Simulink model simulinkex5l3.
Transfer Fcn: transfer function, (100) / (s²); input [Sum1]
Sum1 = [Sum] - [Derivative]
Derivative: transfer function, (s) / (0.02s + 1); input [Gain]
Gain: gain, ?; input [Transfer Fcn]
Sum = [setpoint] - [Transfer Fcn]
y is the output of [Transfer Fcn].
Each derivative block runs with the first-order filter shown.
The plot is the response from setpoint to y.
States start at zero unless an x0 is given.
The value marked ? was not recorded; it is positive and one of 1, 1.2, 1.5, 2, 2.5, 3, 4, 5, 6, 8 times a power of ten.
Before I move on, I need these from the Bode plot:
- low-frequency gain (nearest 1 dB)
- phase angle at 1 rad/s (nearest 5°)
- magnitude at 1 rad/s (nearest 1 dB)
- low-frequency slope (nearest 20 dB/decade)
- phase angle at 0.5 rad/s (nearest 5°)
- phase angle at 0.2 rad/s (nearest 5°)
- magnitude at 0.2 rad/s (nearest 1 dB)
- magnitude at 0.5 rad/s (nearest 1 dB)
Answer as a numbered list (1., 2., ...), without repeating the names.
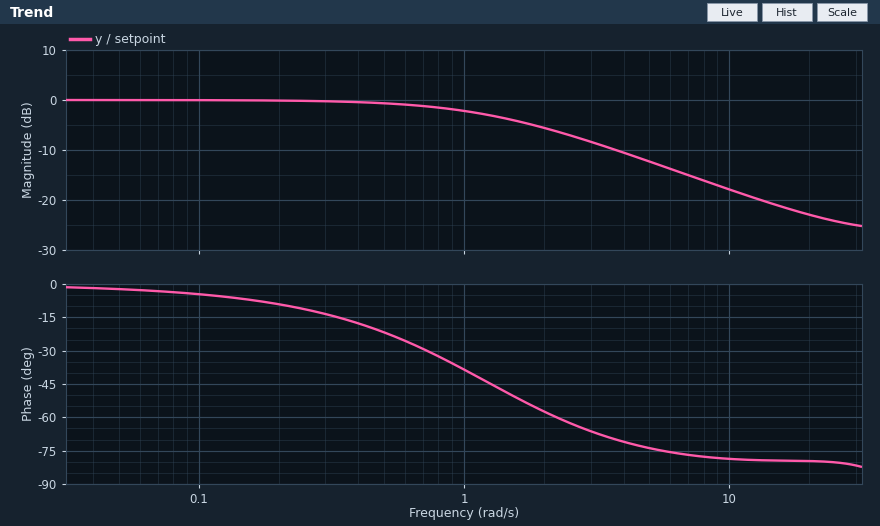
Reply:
1. 0 dB
2. -40°
3. -2 dB
4. 0 dB/decade
5. -20°
6. -10°
7. 0 dB
8. -1 dB
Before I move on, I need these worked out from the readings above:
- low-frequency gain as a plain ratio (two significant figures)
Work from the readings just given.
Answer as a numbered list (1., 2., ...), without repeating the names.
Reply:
1. 1.0
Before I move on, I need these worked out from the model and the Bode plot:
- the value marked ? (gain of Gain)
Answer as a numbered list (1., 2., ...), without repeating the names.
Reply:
1. 0.8
